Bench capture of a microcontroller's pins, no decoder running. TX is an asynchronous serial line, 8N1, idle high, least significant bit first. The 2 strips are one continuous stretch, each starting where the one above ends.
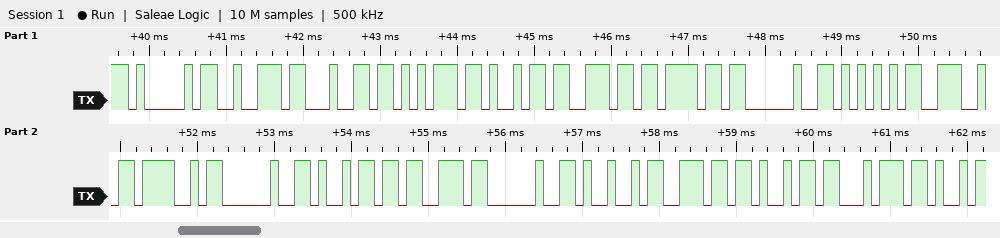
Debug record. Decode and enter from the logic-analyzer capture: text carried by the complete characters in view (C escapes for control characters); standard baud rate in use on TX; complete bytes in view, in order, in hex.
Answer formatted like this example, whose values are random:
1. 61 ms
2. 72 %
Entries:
1. "Arduino UNO is Init"
2. 9600 baud
3. 41 72 64 75 69 6E 6F 20 55 4E 4F 20 69 73 20 49 6E 69 74
